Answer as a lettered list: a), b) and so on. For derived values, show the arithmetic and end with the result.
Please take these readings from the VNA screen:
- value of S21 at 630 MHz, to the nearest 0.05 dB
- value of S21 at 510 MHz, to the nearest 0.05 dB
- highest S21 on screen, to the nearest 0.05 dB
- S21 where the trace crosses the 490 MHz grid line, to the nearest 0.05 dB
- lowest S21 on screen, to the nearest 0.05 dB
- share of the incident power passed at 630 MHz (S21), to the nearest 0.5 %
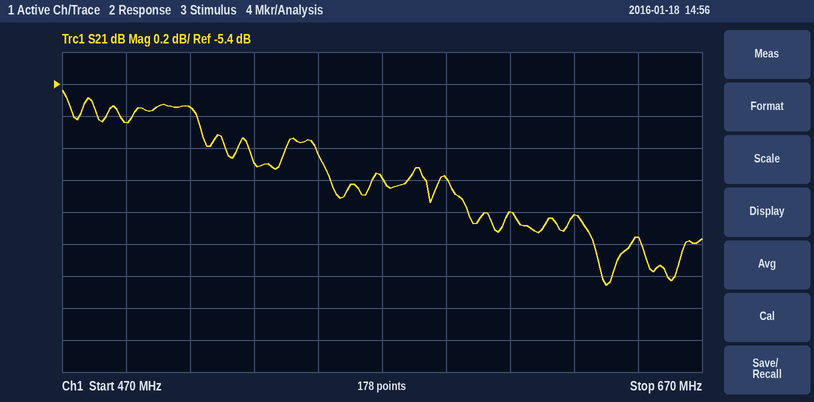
a) -6.20 dB
b) -5.55 dB
c) -5.45 dB
d) -5.65 dB
e) -6.65 dB
f) 10^(-6.2/10) ≈ 24.0 %
